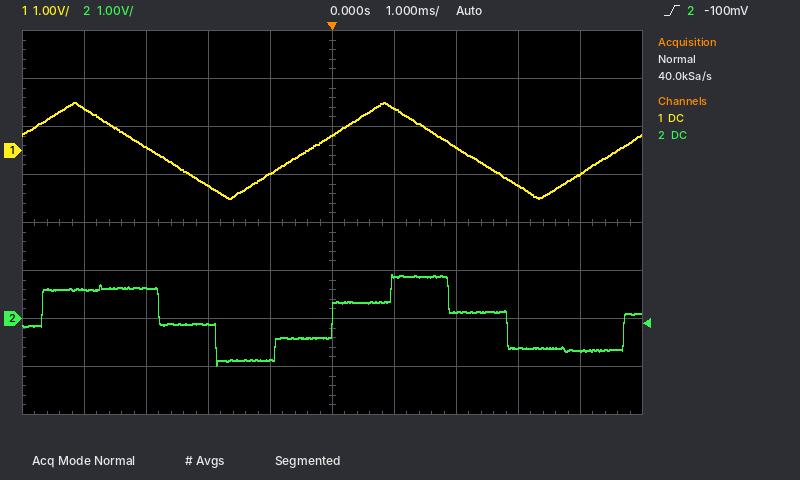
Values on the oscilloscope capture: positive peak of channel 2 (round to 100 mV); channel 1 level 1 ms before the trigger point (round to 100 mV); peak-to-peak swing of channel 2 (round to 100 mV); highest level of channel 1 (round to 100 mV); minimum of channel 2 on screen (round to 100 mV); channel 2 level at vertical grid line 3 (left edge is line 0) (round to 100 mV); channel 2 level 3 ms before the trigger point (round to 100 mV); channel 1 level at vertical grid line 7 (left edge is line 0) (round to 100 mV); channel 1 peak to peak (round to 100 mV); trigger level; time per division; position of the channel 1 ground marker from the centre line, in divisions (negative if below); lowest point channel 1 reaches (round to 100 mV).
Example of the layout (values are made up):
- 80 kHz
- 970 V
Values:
- 900 mV
- -500 mV
- 1.9 V
- 1.0 V
- -1.0 V
- -100 mV
- 600 mV
- 100 mV
- 2.0 V
- -100 mV
- 1 ms
- +1.5 div
- -1.0 V
